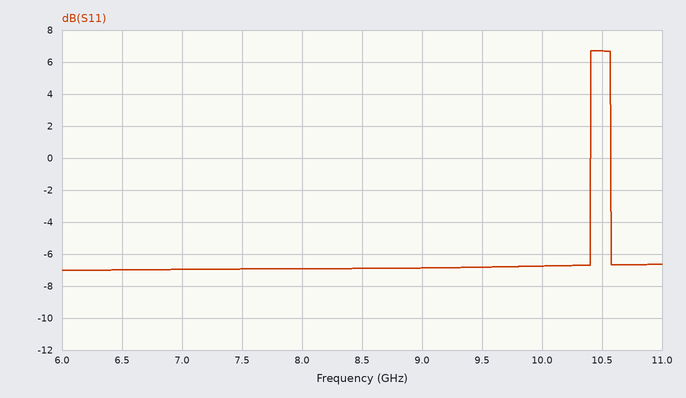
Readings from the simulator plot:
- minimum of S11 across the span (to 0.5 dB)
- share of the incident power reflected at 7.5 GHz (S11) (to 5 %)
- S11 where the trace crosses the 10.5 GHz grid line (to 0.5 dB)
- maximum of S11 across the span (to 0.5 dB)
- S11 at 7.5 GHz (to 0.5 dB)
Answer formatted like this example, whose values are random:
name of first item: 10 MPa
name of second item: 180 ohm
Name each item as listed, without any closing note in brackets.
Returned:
minimum of S11 across the span: -7.0 dB
share of the incident power reflected at 7.5 GHz (S11): 20 %
S11 where the trace crosses the 10.5 GHz grid line: 6.5 dB
maximum of S11 across the span: 6.5 dB
S11 at 7.5 GHz: -7.0 dB
